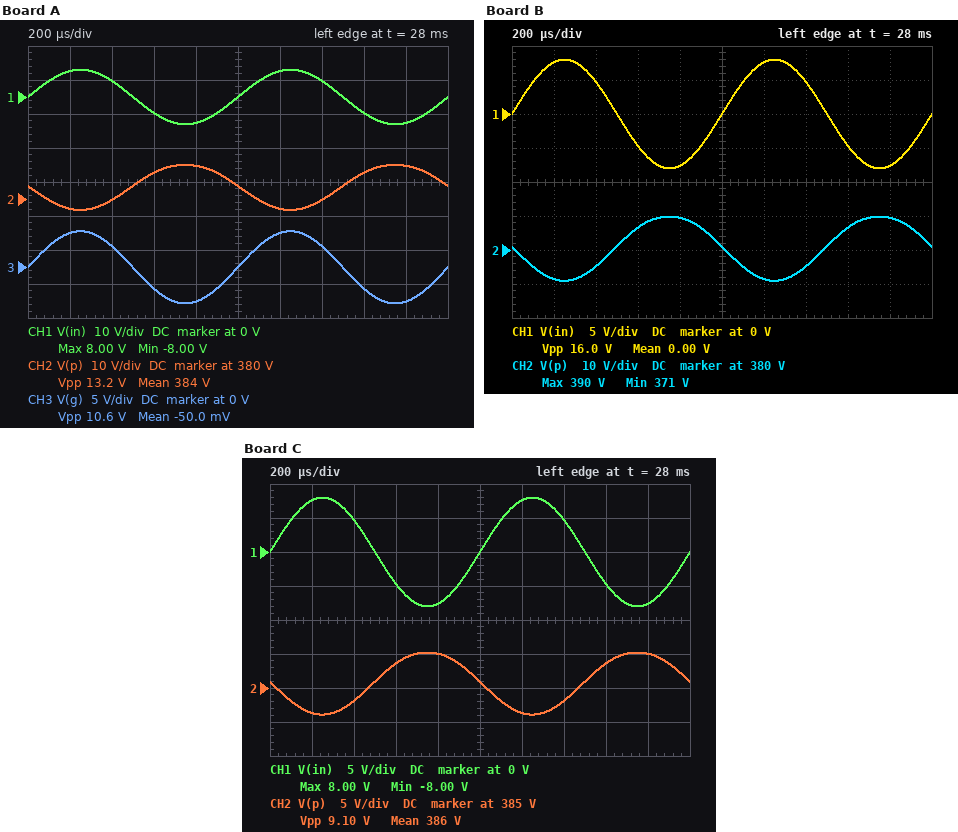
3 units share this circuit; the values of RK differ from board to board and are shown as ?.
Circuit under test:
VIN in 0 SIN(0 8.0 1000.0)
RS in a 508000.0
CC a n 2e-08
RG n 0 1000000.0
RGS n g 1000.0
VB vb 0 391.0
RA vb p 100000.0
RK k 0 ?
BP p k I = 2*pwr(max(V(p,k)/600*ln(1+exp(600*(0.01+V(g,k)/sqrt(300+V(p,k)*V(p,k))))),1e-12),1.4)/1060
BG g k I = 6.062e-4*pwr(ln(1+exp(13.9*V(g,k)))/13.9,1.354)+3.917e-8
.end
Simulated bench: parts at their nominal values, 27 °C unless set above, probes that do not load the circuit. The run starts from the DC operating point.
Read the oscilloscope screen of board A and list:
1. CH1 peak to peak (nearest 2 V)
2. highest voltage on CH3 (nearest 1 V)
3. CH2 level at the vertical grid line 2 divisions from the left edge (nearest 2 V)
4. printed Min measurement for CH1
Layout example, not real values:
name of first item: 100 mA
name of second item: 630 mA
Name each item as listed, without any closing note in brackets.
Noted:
CH1 peak to peak: 16 V
highest voltage on CH3: 5 V
CH2 level at the vertical grid line 2 divisions from the left edge: 380 V
printed Min measurement for CH1: -8.00 V
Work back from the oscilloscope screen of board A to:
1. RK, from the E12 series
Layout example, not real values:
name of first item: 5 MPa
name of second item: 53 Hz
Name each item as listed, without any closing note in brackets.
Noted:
RK, from the E12 series: 68 kΩ
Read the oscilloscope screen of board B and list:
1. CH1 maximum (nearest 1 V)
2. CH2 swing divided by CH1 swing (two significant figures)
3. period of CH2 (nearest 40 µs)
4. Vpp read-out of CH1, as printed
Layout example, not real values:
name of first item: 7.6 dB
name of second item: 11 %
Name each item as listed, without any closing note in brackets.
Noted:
CH1 maximum: 8 V
CH2 swing divided by CH1 swing: 1.2
period of CH2: 1.00 ms
Vpp read-out of CH1, as printed: 16.0 V
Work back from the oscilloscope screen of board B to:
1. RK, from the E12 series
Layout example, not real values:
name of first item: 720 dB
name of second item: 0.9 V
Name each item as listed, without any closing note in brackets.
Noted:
RK, from the E12 series: 47 kΩ
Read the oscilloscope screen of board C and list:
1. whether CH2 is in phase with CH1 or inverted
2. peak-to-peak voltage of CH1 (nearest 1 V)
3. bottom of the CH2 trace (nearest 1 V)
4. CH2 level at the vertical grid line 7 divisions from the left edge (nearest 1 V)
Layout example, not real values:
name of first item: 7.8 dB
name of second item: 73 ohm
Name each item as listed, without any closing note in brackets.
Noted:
whether CH2 is in phase with CH1 or inverted: inverted
peak-to-peak voltage of CH1: 16 V
bottom of the CH2 trace: 381 V
CH2 level at the vertical grid line 7 divisions from the left edge: 383 V
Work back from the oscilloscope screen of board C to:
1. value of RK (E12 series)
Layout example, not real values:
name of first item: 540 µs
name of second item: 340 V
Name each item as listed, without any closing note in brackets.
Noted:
value of RK: 100 kΩ
